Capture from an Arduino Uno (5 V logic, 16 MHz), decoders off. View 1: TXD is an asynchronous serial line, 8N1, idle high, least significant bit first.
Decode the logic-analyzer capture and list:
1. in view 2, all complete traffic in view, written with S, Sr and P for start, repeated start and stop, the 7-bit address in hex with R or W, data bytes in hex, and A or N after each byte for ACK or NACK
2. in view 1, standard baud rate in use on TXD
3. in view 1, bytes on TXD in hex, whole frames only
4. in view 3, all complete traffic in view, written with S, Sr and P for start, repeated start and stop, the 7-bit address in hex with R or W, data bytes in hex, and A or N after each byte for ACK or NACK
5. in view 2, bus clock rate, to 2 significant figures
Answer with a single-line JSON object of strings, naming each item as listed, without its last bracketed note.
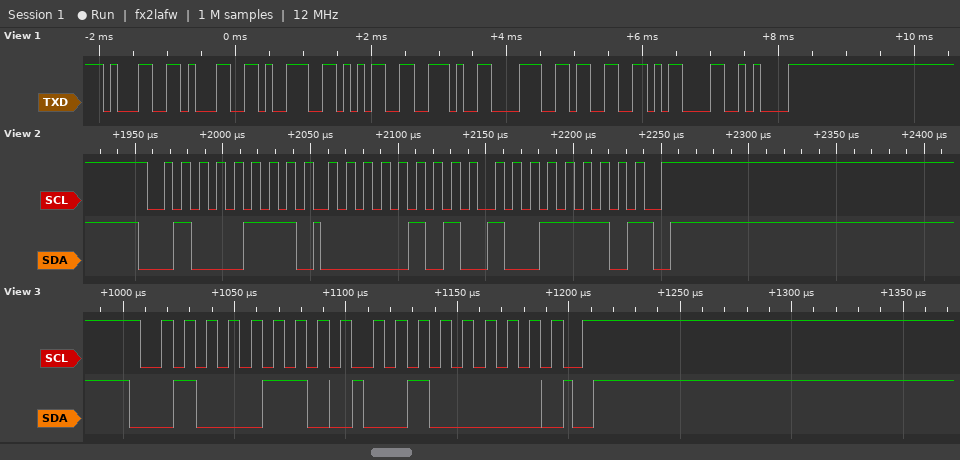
{"in view 2, all complete traffic in view, written with S, Sr and P for start, repeated start and stop, the 7-bit address in hex with R or W, data bytes in hex, and A or N after each byte for ACK or NACK": "S 23R A 05 A 9E N P", "in view 1, standard baud rate in use on TXD": "9600 baud", "in view 1, bytes on TXD in hex, whole frames only": "31 31 39 35 2E 38 33 0D 0A", "in view 3, all complete traffic in view, written with S, Sr and P for start, repeated start and stop, the 7-bit address in hex with R or W, data bytes in hex, and A or N after each byte for ACK or NACK": "S 23W A 20 A P", "in view 2, bus clock rate, to 2 significant figures": "100 kHz"}
